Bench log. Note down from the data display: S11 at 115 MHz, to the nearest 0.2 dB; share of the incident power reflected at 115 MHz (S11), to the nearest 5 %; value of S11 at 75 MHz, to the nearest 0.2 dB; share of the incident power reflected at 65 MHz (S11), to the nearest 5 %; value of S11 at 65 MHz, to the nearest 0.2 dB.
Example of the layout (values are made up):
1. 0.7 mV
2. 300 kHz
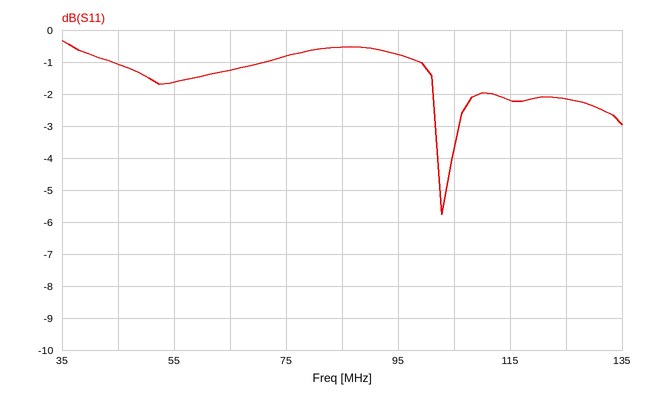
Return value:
1. -2.2 dB
2. 60 %
3. -0.8 dB
4. 75 %
5. -1.2 dB
